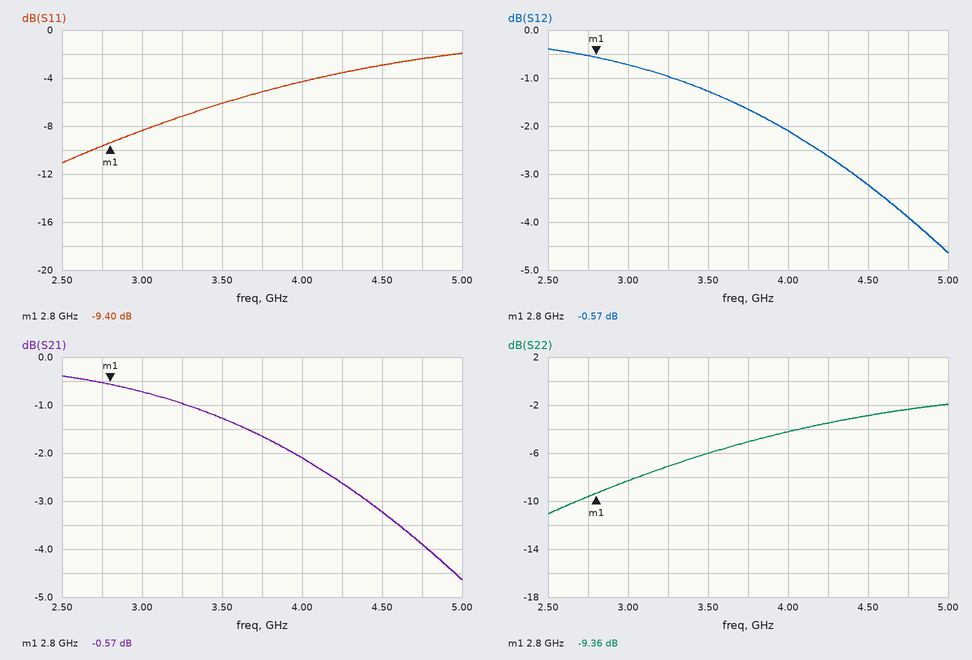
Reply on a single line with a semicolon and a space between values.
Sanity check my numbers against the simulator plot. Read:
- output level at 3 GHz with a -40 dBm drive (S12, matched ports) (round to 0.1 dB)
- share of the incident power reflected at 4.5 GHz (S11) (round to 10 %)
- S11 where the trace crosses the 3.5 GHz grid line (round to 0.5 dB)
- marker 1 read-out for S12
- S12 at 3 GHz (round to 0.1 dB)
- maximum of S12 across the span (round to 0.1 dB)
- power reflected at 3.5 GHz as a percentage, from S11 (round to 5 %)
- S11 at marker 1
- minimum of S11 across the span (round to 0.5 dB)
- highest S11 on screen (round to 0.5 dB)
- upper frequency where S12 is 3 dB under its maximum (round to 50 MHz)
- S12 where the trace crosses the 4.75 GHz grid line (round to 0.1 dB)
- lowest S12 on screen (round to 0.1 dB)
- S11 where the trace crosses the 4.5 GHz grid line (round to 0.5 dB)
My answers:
-40.7 dBm; 50 %; -6.0 dB; -0.57 dB; -0.7 dB; -0.4 dB; 25 %; -9.40 dB; -11.0 dB; -2.0 dB; 4.55 GHz; -3.9 dB; -4.6 dB; -3.0 dB
